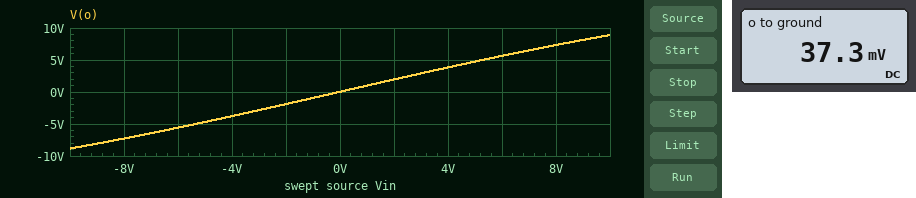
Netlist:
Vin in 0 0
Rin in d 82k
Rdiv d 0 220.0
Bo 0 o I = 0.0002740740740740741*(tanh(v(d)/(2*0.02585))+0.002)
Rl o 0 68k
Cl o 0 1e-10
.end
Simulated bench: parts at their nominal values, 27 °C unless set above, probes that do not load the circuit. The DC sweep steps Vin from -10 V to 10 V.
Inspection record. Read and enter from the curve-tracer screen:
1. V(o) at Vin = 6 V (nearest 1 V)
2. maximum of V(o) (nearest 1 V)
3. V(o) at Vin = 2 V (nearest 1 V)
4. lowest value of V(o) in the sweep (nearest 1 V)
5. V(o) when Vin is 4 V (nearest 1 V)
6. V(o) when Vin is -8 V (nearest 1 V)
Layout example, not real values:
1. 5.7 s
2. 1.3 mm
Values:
1. 6 V
2. 9 V
3. 2 V
4. -9 V
5. 4 V
6. -7 V
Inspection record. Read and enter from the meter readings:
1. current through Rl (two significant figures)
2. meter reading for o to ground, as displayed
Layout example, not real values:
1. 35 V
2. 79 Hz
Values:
1. 550 nA
2. 37.3 mV
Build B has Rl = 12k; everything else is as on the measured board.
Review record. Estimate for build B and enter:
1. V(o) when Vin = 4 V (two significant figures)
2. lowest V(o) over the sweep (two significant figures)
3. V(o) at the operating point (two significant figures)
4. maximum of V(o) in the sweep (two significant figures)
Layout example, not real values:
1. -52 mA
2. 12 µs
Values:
1. 680 mV
2. -1.6 V
3. 6.6 mV
4. 1.6 V
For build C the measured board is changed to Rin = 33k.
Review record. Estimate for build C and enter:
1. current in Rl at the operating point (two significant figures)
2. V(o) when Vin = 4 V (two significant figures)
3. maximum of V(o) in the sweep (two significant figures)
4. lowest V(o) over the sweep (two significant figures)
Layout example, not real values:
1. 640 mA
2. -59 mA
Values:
1. 550 nA
2. 8.8 V
3. 16 V
4. -16 V
